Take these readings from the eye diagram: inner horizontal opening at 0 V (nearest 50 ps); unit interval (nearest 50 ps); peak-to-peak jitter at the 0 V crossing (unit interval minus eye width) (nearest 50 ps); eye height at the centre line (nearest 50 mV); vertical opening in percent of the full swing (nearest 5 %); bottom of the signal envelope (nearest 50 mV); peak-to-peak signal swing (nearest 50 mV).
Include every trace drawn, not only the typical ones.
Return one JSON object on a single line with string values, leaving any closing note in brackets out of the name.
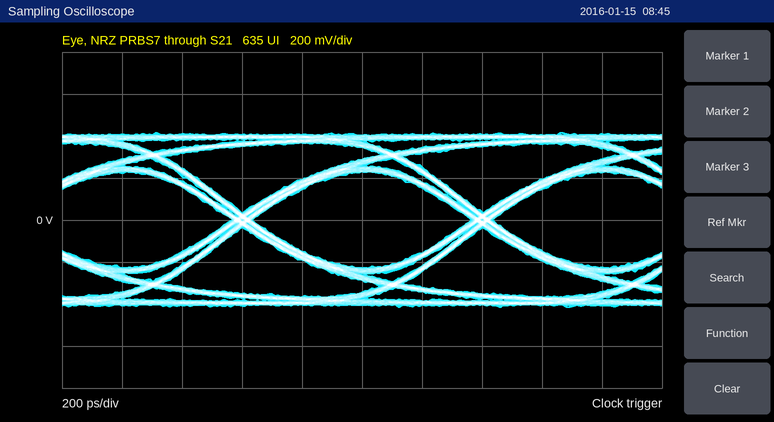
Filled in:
{"inner horizontal opening at 0 V": "750 ps", "unit interval": "800 ps", "peak-to-peak jitter at the 0 V crossing (unit interval minus eye width)": "50 ps", "eye height at the centre line": "450 mV", "vertical opening in percent of the full swing": "55 %", "bottom of the signal envelope": "-400 mV", "peak-to-peak signal swing": "850 mV"}
